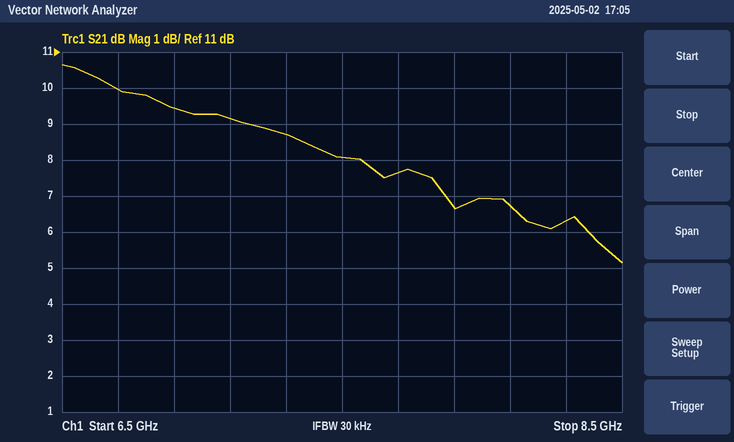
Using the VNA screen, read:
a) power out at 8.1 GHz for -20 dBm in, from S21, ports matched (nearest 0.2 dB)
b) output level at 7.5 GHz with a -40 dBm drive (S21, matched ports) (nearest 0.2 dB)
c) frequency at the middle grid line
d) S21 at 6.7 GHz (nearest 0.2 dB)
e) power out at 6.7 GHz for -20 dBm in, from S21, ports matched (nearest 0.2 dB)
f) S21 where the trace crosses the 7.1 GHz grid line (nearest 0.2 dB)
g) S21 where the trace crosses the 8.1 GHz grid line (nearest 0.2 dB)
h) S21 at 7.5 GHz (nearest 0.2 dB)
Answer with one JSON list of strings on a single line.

["-13.2 dBm", "-32.0 dBm", "7.5 GHz", "10.0 dB", "-10.0 dBm", "9.2 dB", "6.8 dB", "8.0 dB"]
